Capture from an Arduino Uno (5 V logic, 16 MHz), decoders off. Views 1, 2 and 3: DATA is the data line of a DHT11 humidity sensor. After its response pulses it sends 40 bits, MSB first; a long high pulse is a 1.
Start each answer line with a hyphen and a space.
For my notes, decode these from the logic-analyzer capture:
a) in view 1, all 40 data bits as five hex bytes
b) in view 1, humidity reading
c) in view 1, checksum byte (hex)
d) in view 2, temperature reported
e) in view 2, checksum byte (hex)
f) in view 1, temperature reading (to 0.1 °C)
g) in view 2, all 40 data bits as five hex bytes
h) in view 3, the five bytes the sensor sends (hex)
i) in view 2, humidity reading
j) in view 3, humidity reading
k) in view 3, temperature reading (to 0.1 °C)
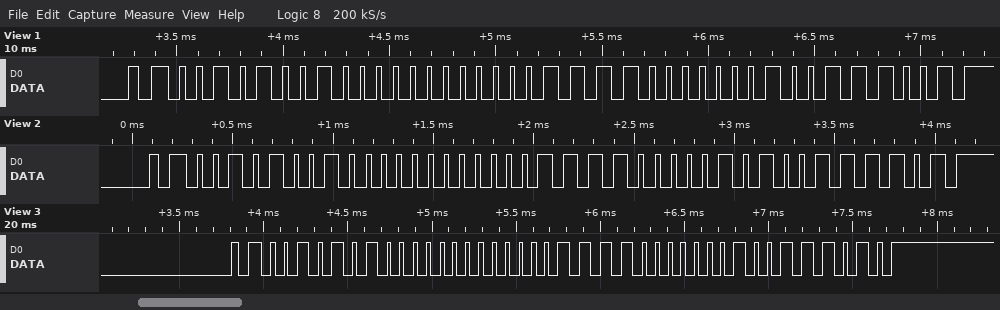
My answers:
- 29 00 0F 01 39
- 41 %
- 0x39
- 15.5 °C
- 0x3D
- 15.1 °C
- 29 00 0F 05 3D
- 2A 00 0F 01 3A
- 41 %
- 42 %
- 15.1 °C
